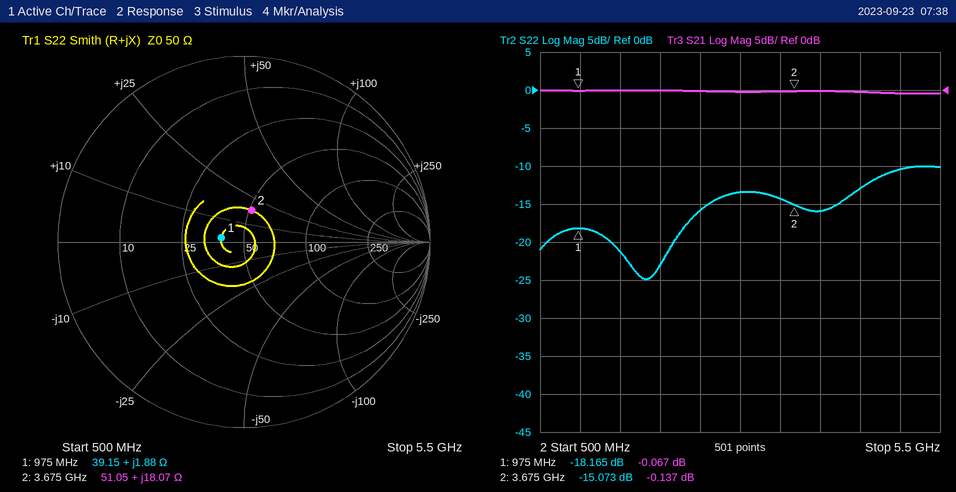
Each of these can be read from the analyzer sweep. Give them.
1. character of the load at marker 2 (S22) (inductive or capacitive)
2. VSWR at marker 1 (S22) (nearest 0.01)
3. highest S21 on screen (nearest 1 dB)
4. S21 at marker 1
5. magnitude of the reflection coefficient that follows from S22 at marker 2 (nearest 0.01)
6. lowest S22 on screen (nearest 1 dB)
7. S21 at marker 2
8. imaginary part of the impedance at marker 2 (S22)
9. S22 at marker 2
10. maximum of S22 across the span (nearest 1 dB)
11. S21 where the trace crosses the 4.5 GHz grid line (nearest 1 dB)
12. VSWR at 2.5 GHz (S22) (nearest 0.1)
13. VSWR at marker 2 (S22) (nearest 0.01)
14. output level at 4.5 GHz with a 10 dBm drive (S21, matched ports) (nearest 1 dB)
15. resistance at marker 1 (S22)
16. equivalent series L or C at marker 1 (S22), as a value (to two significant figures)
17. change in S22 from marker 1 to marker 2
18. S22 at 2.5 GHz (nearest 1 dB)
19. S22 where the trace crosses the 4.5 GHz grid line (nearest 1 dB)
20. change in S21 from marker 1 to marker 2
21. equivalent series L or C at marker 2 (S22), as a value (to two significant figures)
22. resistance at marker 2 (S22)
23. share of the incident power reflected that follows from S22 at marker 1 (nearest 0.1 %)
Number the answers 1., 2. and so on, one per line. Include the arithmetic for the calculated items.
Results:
1. inductive
2. 1.28
3. 0 dB
4. -0.067 dB
5. 10^(-15.073/20) ≈ 0.18
6. -25 dB
7. -0.137 dB
8. +18.07 Ω
9. -15.073 dB
10. -10 dB
11. 0 dB
12. |Γ| = 10^(-16/20) = 0.1585; VSWR = (1 + 0.1585)/(1 − 0.1585) ≈ 1.4
13. 1.43
14. 10 dBm + (0 dB) = 10 dBm
15. 39.15 Ω
16. L = 1.88 Ω/(2π × 975 MHz) ≈ 307 pH, so 310 pH to two significant figures
17. -15.073 − (-18.165) = 3.092 dB
18. -16 dB
19. -13 dB
20. -0.137 − (-0.067) = -0.070 dB
21. L = 18.07 Ω/(2π × 3.675 GHz) ≈ 783 pH, so 780 pH to two significant figures
22. 51.05 Ω
23. 10^(-18.165/10) ≈ 1.5 %
